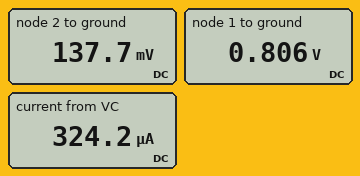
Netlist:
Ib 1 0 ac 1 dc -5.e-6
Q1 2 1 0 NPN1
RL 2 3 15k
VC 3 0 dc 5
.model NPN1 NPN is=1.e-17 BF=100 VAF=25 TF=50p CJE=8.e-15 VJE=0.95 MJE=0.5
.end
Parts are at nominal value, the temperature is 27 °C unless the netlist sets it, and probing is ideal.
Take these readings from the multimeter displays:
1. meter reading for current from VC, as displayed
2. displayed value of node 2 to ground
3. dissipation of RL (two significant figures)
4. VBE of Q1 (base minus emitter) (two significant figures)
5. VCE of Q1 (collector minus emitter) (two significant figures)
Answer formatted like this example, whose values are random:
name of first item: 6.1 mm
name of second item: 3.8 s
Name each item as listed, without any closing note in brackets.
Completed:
meter reading for current from VC, as displayed: 324.2 µA
displayed value of node 2 to ground: 137.7 mV
dissipation of RL: 1.6 mW
VBE of Q1 (base minus emitter): 810 mV
VCE of Q1 (collector minus emitter): 140 mV
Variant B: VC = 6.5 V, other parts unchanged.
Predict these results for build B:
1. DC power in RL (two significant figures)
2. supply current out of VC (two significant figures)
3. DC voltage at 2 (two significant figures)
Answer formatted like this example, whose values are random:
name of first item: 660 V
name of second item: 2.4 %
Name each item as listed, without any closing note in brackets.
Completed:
DC power in RL: 2.7 mW
supply current out of VC: 420 µA
DC voltage at 2: 170 mV
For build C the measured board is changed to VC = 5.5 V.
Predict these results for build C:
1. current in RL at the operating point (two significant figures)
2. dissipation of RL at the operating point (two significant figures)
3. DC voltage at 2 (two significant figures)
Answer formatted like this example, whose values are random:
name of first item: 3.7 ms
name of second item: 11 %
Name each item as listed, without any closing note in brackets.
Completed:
current in RL at the operating point: 360 µA
dissipation of RL at the operating point: 1.9 mW
DC voltage at 2: 150 mV
